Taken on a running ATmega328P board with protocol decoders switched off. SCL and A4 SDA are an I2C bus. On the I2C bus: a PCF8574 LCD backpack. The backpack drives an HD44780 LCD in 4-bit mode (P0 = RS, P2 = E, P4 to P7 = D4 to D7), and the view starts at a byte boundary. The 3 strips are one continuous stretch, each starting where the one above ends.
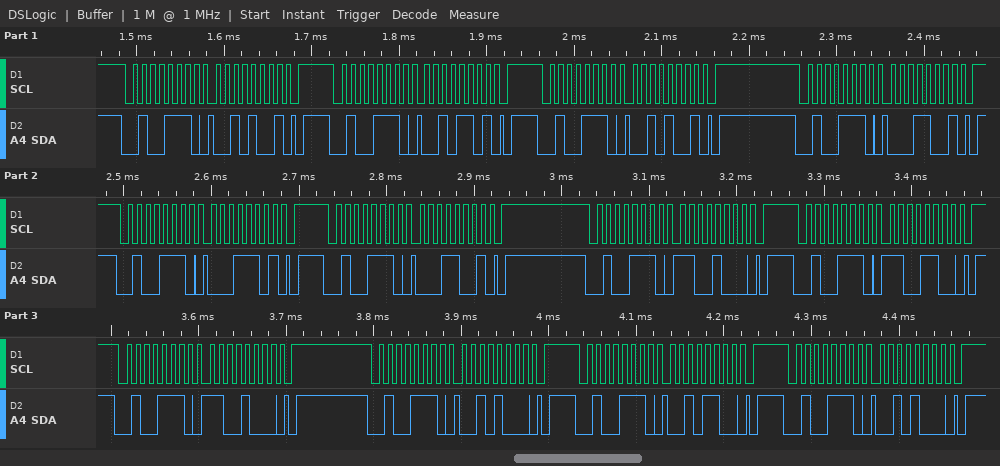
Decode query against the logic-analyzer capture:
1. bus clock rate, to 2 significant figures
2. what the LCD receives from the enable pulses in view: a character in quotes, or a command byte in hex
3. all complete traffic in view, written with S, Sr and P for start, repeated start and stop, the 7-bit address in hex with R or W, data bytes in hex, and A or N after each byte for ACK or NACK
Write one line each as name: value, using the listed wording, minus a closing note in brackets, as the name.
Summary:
bus clock rate, to 2 significant figures: 100 kHz
what the LCD receives from the enable pulses in view: a character in quotes, or a command byte in hex: '!' 0xC2
all complete traffic in view, written with S, Sr and P for start, repeated start and stop, the 7-bit address in hex with R or W, data bytes in hex, and A or N after each byte for ACK or NACK: S 27W A 29 A P S 27W A 2D A P S 27W A 29 A P S 27W A 19 A P S 27W A 1D A P S 27W A 19 A P S 27W A C8 A P S 27W A CC A P S 27W A C8 A P S 27W A 28 A P S 27W A 2C A P S 27W A 28 A P
